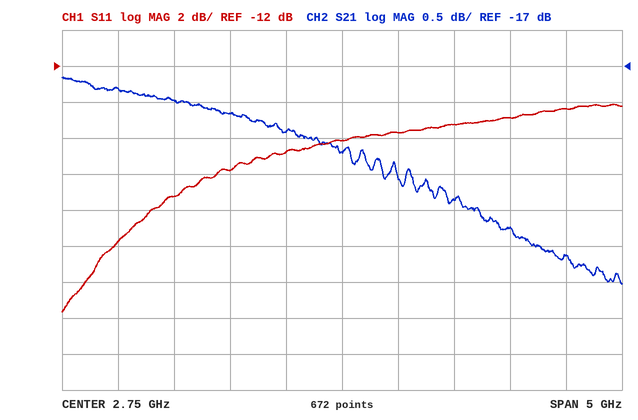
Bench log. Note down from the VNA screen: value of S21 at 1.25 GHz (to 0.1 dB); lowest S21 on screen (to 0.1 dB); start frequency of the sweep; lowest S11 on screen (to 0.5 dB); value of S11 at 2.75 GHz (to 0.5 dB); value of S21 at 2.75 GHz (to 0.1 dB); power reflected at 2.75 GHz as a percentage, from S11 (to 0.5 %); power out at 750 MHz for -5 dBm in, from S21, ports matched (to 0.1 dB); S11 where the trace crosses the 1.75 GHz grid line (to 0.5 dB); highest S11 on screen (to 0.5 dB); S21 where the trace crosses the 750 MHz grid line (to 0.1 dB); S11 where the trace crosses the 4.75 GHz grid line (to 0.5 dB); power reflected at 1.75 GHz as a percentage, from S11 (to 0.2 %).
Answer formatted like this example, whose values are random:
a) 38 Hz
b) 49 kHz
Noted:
a) -17.5 dB
b) -20.0 dB
c) 250 MHz
d) -25.5 dB
e) -16.0 dB
f) -18.2 dB
g) 2.5 %
h) -22.3 dBm
i) -18.0 dB
j) -14.0 dB
k) -17.3 dB
l) -14.5 dB
m) 1.6 %
